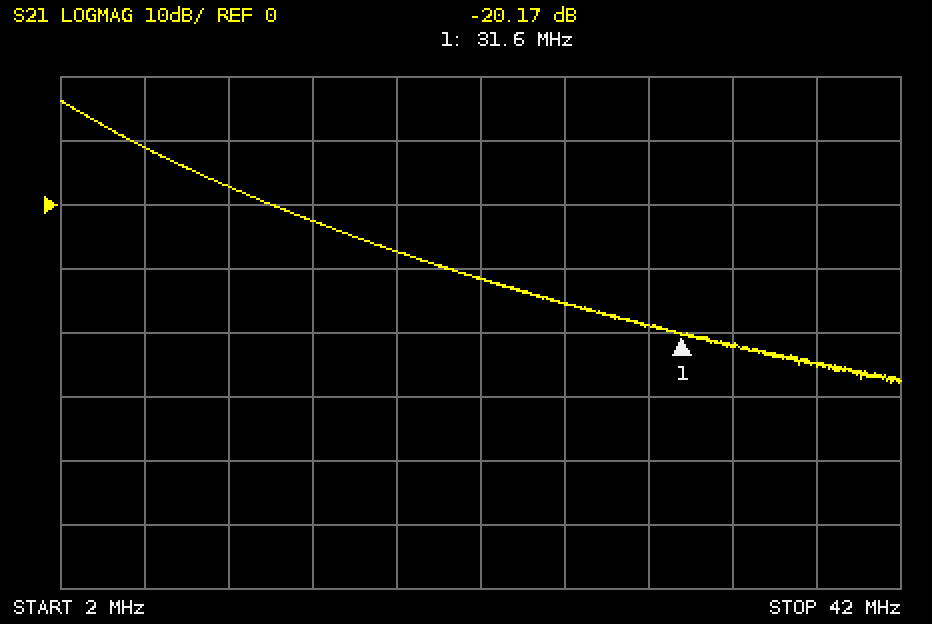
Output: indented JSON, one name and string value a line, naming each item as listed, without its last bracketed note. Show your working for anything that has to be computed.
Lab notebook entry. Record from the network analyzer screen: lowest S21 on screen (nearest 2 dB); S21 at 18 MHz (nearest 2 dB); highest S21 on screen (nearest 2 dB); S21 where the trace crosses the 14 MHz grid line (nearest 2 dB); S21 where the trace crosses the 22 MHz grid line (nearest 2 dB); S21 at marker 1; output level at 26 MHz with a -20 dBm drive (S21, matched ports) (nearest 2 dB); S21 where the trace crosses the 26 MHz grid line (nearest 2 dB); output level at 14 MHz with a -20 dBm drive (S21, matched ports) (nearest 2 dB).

{
  "lowest S21 on screen": "-28 dB",
  "S21 at 18 MHz": "-8 dB",
  "highest S21 on screen": "16 dB",
  "S21 where the trace crosses the 14 MHz grid line": "-2 dB",
  "S21 where the trace crosses the 22 MHz grid line": "-12 dB",
  "S21 at marker 1": "-20.17 dB",
  "output level at 26 MHz with a -20 dBm drive (S21, matched ports)": "-20 dBm + (-16 dB) = -36 dBm",
  "S21 where the trace crosses the 26 MHz grid line": "-16 dB",
  "output level at 14 MHz with a -20 dBm drive (S21, matched ports)": "-20 dBm + (-2 dB) = -22 dBm"
}
